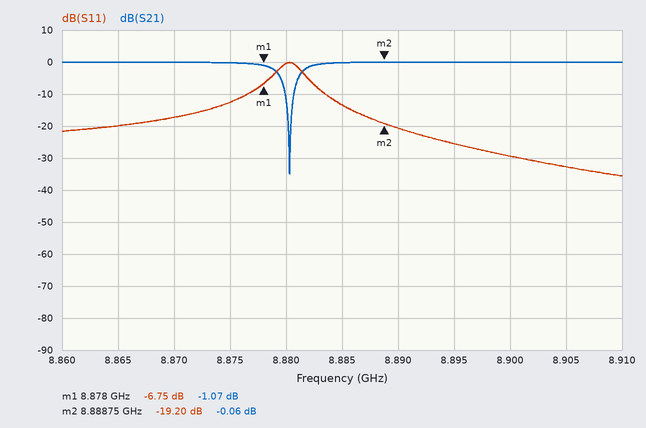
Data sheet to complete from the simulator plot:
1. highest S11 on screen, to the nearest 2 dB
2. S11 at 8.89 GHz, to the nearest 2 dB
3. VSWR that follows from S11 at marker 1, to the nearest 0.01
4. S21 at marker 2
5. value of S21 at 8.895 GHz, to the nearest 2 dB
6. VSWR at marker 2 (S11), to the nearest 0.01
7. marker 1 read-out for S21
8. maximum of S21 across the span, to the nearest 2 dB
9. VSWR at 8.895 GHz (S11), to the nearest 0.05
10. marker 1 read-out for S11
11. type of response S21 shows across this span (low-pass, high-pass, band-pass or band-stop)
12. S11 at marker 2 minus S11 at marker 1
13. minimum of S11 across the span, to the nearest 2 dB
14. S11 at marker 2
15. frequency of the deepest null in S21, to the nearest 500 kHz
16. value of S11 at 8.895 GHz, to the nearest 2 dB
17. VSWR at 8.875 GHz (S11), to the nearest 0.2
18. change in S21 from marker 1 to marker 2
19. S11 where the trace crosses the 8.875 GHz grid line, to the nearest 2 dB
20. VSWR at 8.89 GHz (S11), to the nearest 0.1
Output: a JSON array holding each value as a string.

["0 dB", "-20 dB", "2.70", "-0.06 dB", "0 dB", "1.25", "-1.07 dB", "0 dB", "1.10", "-6.75 dB", "band-stop", "-12.45 dB", "-36 dB", "-19.20 dB", "8.8805 GHz", "-26 dB", "1.6", "1.01 dB", "-12 dB", "1.2"]
